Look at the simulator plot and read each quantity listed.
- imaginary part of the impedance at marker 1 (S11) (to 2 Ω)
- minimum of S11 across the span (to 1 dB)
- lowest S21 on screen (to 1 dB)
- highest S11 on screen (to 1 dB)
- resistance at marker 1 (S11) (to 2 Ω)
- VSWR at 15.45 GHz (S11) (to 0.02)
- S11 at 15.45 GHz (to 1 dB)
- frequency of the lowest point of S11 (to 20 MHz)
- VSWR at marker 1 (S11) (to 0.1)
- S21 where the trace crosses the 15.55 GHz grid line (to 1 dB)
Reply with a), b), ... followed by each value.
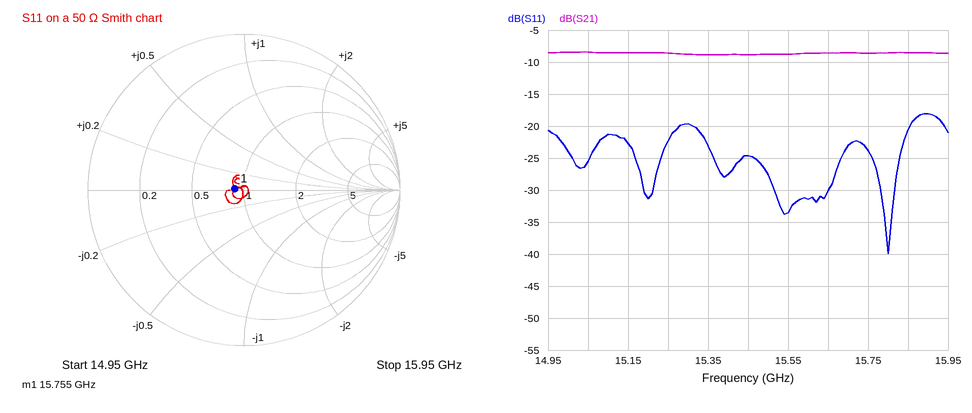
a) 0 Ω
b) -40 dB
c) -9 dB
d) -18 dB
e) 44 Ω
f) 1.12
g) -25 dB
h) 15.80 GHz
i) 1.1
j) -9 dB
